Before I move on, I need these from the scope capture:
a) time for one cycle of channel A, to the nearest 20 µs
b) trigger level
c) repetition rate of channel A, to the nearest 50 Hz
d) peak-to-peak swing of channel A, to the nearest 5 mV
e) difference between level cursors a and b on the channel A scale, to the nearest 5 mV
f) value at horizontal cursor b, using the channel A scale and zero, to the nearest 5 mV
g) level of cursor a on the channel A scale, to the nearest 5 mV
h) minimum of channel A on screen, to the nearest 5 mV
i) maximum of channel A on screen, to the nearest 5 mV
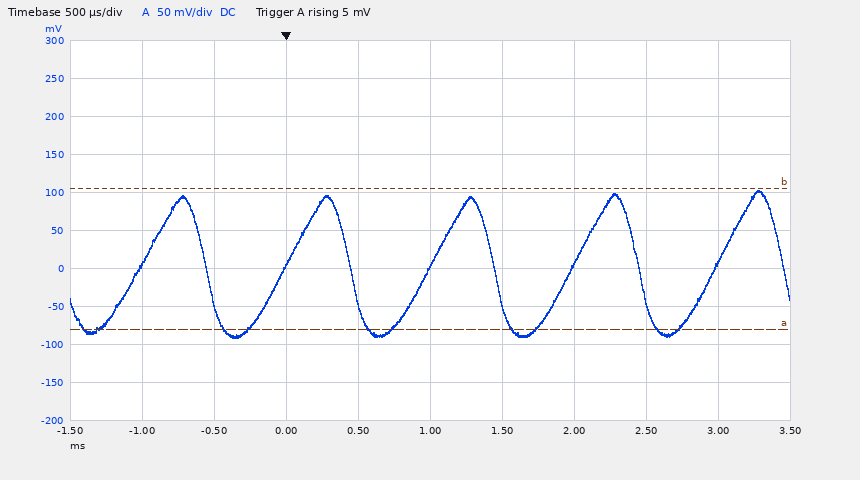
1.00 ms
5 mV
1.00 kHz
195 mV
185 mV
105 mV
-80 mV
-90 mV
105 mV
